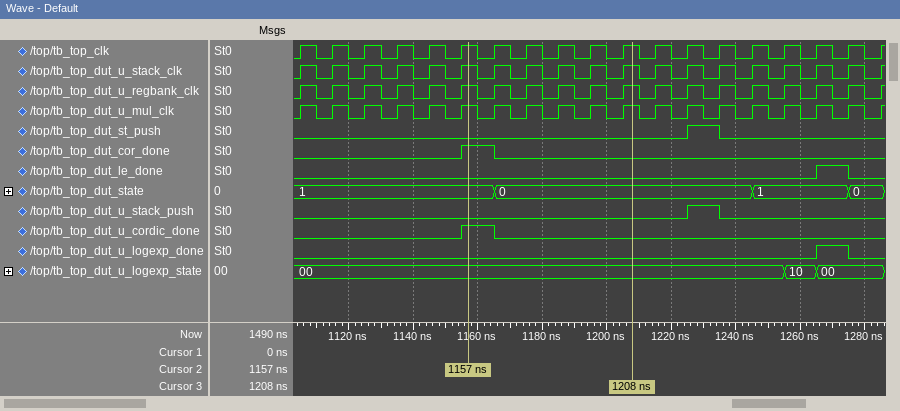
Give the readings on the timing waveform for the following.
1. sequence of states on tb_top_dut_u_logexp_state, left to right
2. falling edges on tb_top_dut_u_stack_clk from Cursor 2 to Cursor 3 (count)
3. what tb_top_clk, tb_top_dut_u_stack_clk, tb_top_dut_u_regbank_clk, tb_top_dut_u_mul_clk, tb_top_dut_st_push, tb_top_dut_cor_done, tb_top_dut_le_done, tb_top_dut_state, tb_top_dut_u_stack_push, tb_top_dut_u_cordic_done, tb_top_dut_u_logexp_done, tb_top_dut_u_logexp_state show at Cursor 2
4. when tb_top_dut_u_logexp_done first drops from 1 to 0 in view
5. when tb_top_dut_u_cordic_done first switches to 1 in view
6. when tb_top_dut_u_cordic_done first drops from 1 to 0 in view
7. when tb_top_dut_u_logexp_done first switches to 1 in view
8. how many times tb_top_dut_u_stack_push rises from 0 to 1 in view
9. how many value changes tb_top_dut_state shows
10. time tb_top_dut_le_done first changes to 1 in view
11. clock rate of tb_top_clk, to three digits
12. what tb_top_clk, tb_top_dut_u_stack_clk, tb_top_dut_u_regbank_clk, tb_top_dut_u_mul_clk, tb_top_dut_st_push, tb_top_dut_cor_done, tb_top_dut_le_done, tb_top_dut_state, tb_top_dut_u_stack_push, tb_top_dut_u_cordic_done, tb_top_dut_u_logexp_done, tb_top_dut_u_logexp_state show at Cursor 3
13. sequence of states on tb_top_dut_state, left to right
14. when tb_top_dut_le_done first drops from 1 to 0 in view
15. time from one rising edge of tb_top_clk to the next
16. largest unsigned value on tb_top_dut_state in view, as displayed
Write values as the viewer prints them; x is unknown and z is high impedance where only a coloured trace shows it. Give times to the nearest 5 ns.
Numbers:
00, 10, 00
5
tb_top_clk=1, tb_top_dut_u_stack_clk=1, tb_top_dut_u_regbank_clk=1, tb_top_dut_u_mul_clk=1, tb_top_dut_st_push=0, tb_top_dut_cor_done=1, tb_top_dut_le_done=0, tb_top_dut_state=1, tb_top_dut_u_stack_push=0, tb_top_dut_u_cordic_done=1, tb_top_dut_u_logexp_done=0, tb_top_dut_u_logexp_state=00
1275 ns
1155 ns
1165 ns
1265 ns
1
3
1265 ns
100 MHz
tb_top_clk=1, tb_top_dut_u_stack_clk=1, tb_top_dut_u_regbank_clk=1, tb_top_dut_u_mul_clk=1, tb_top_dut_st_push=0, tb_top_dut_cor_done=0, tb_top_dut_le_done=0, tb_top_dut_state=0, tb_top_dut_u_stack_push=0, tb_top_dut_u_cordic_done=0, tb_top_dut_u_logexp_done=0, tb_top_dut_u_logexp_state=00
1, 0, 1, 0
1275 ns
10 ns
1
